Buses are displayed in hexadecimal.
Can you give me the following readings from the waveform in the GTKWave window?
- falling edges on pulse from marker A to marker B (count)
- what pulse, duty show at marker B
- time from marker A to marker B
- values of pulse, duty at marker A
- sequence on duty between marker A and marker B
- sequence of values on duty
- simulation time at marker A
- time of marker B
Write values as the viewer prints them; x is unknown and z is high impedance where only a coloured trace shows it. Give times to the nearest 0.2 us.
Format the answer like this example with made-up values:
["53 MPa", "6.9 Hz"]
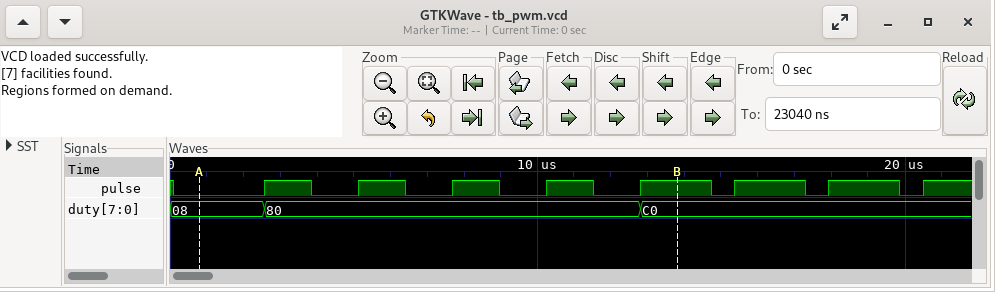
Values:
["4", "pulse=1, duty=C0", "13 us", "pulse=0, duty=08", "08, 80, C0", "08, 80, C0", "0.8 us", "13.8 us"]
